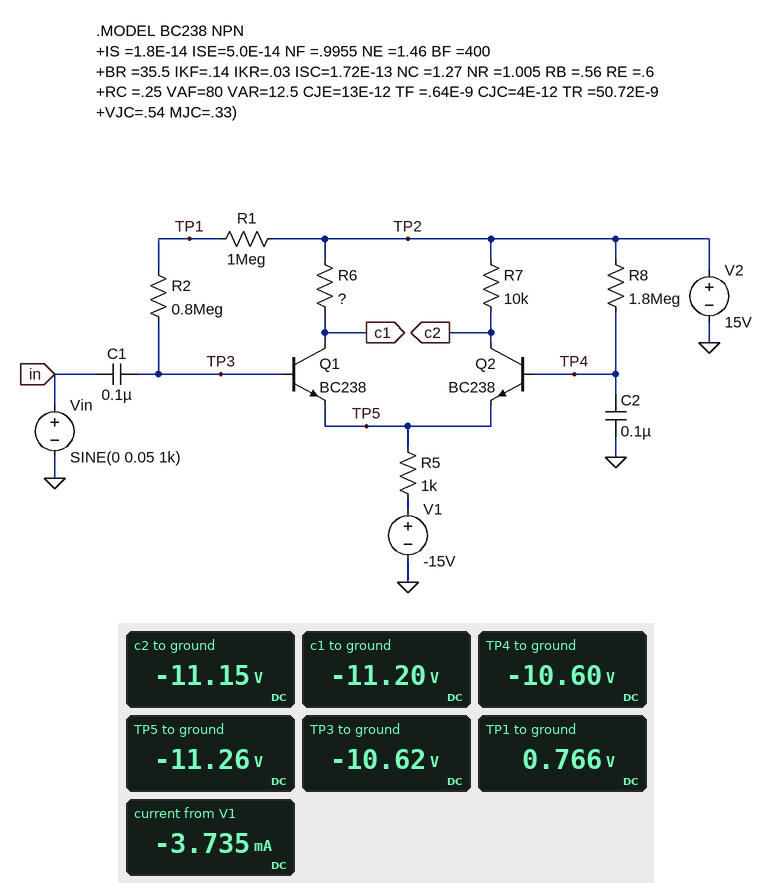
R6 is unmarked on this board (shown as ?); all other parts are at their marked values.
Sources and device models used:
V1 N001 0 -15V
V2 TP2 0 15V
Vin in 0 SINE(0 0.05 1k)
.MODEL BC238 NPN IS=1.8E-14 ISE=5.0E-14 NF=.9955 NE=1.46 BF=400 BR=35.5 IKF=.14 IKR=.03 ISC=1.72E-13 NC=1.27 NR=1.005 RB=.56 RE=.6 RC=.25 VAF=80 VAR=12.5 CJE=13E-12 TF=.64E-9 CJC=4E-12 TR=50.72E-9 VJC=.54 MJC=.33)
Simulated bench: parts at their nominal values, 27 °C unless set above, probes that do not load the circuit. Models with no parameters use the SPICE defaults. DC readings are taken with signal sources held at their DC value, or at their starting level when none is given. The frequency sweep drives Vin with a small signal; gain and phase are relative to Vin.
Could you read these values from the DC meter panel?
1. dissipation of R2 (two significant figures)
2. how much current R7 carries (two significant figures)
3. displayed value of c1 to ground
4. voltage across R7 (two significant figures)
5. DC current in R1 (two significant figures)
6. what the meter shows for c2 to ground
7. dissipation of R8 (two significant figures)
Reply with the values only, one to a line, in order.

160 µW
2.6 mA
-11.20 V
26 V
14 µA
-11.15 V
360 µW
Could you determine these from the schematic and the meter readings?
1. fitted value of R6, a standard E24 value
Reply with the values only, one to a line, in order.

24 kΩ
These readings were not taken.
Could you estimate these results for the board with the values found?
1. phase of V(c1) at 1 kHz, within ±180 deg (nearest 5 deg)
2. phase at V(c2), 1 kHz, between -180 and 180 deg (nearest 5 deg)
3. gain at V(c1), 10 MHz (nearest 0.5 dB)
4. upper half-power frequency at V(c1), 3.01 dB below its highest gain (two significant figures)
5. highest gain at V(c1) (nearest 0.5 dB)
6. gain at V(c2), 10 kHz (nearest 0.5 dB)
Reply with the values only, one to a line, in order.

-100 deg
100 deg
8.0 dB
2.4 MHz
19.0 dB
20.0 dB
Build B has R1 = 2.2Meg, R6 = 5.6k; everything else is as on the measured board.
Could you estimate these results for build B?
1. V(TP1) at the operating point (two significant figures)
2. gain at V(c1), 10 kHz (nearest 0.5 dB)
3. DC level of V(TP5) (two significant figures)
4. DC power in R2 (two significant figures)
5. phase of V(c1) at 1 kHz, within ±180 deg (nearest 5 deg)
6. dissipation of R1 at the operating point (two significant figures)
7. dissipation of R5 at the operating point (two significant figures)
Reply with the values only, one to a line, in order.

-2.8 V
33.5 dB
-9.9 V
52 µW
-140 deg
140 µW
26 mW
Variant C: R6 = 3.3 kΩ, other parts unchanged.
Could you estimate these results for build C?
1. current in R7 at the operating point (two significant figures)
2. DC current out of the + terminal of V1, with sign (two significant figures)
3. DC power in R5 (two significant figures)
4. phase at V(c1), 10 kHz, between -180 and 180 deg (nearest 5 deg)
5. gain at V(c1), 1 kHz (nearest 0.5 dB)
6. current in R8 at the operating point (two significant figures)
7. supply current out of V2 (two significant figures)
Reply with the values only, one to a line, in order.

2.3 mA
-6.5 mA
42 mW
-135 deg
14.0 dB
13 µA
6.5 mA
